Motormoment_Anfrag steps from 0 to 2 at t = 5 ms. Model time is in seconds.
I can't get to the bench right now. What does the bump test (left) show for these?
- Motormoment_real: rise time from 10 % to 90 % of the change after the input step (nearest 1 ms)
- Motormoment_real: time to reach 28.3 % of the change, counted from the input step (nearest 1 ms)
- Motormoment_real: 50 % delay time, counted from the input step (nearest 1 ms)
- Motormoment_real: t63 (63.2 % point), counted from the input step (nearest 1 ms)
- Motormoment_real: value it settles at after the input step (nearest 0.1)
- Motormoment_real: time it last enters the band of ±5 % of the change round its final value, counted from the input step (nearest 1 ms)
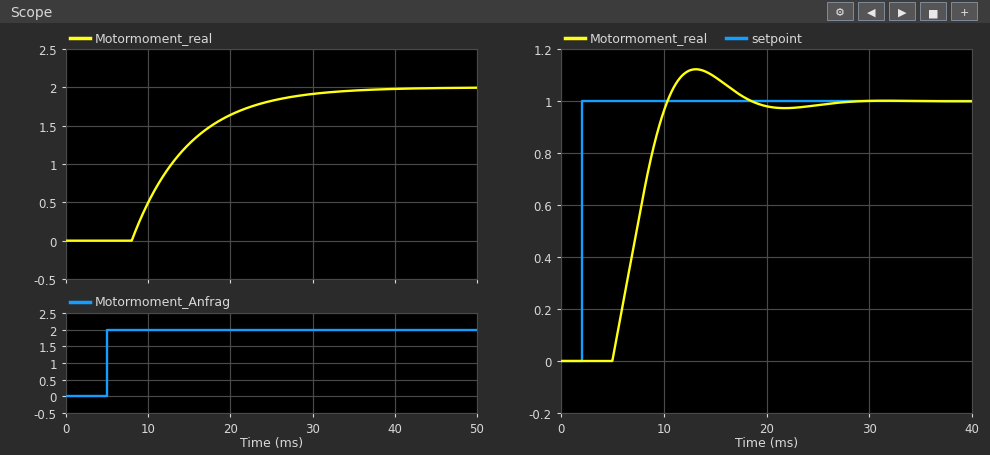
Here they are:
15 ms
5 ms
8 ms
10 ms
2.0
24 ms
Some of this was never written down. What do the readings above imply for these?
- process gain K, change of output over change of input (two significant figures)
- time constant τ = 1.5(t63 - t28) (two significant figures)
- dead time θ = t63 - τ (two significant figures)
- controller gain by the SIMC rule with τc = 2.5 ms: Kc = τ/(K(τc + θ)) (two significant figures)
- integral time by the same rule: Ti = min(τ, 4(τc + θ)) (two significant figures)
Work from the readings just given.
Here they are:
1.0
7.5 ms
2.5 ms
1.5
7.5 ms
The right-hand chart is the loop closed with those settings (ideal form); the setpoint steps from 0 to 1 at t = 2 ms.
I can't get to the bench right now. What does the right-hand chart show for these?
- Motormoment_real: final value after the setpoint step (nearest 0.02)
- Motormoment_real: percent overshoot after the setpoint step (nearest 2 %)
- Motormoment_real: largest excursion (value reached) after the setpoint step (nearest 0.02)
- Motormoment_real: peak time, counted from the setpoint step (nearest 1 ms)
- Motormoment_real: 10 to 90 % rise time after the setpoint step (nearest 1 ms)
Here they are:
1.00
12 %
1.12
11 ms
4 ms
